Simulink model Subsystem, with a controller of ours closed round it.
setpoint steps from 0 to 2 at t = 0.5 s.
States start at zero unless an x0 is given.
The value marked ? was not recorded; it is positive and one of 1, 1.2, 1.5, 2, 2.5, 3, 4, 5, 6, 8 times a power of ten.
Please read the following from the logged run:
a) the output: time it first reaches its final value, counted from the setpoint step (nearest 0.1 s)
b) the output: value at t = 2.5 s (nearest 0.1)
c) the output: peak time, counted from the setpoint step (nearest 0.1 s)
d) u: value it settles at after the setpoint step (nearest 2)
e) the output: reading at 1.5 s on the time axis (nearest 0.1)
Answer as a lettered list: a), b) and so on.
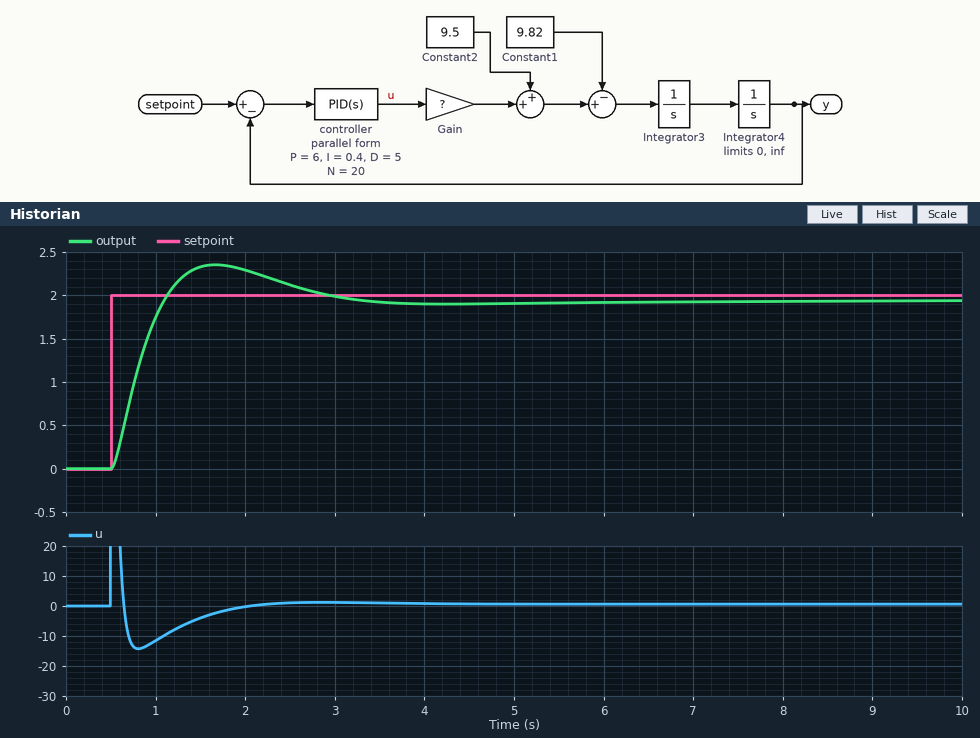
a) 0.6 s
b) 2.1
c) 1.2 s
d) 0
e) 2.3
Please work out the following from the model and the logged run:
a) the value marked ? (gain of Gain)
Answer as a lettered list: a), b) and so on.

a) 0.5
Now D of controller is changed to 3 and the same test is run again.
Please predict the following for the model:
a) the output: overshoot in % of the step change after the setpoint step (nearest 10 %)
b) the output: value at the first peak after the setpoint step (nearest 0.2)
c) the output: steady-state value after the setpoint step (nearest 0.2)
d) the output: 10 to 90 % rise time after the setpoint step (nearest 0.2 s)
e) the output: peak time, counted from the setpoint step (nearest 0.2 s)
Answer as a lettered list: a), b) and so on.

a) 30 %
b) 2.6
c) 2.0
d) 0.6 s
e) 1.4 s
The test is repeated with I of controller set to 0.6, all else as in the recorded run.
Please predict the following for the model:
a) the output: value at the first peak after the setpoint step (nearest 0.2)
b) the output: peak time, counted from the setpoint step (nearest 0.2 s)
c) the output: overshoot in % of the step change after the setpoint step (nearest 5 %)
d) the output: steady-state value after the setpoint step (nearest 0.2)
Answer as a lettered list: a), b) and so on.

a) 2.4
b) 1.2 s
c) 20 %
d) 2.0
